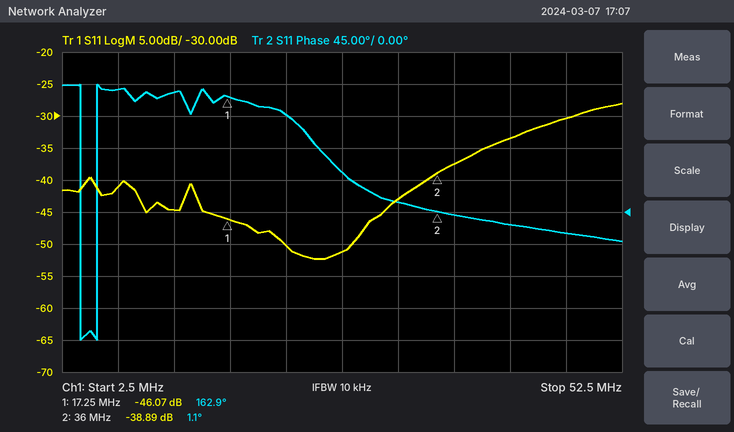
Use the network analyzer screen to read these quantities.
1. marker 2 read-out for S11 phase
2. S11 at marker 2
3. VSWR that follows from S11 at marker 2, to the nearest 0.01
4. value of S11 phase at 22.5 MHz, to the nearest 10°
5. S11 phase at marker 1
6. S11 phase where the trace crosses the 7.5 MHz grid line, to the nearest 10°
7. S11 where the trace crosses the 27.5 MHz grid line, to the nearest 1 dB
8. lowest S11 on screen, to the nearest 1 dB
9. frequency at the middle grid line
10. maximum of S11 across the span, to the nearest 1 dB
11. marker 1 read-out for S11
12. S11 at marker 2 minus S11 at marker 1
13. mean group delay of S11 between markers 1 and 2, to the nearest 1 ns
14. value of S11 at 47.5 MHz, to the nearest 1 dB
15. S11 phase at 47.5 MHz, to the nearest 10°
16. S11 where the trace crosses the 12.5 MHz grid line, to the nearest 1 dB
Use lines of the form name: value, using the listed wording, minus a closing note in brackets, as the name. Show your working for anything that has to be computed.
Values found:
marker 2 read-out for S11 phase: 1.1°
S11 at marker 2: -38.89 dB
VSWR that follows from S11 at marker 2, to the nearest 0.01: (1 + 0.0114)/(1 − 0.0114) ≈ 1.02
value of S11 phase at 22.5 MHz, to the nearest 10°: 140°
S11 phase at marker 1: 162.9°
S11 phase where the trace crosses the 7.5 MHz grid line, to the nearest 10°: 170°
S11 where the trace crosses the 27.5 MHz grid line, to the nearest 1 dB: -51 dB
lowest S11 on screen, to the nearest 1 dB: -52 dB
frequency at the middle grid line: 27.5 MHz
maximum of S11 across the span, to the nearest 1 dB: -28 dB
marker 1 read-out for S11: -46.07 dB
S11 at marker 2 minus S11 at marker 1: -38.89 − (-46.07) = 7.18 dB
mean group delay of S11 between markers 1 and 2, to the nearest 1 ns: −(1.1° − (162.9°))/(360° × 18.75 MHz) ≈ 24 ns
value of S11 at 47.5 MHz, to the nearest 1 dB: -30 dB
S11 phase at 47.5 MHz, to the nearest 10°: -30°
S11 where the trace crosses the 12.5 MHz grid line, to the nearest 1 dB: -45 dB
